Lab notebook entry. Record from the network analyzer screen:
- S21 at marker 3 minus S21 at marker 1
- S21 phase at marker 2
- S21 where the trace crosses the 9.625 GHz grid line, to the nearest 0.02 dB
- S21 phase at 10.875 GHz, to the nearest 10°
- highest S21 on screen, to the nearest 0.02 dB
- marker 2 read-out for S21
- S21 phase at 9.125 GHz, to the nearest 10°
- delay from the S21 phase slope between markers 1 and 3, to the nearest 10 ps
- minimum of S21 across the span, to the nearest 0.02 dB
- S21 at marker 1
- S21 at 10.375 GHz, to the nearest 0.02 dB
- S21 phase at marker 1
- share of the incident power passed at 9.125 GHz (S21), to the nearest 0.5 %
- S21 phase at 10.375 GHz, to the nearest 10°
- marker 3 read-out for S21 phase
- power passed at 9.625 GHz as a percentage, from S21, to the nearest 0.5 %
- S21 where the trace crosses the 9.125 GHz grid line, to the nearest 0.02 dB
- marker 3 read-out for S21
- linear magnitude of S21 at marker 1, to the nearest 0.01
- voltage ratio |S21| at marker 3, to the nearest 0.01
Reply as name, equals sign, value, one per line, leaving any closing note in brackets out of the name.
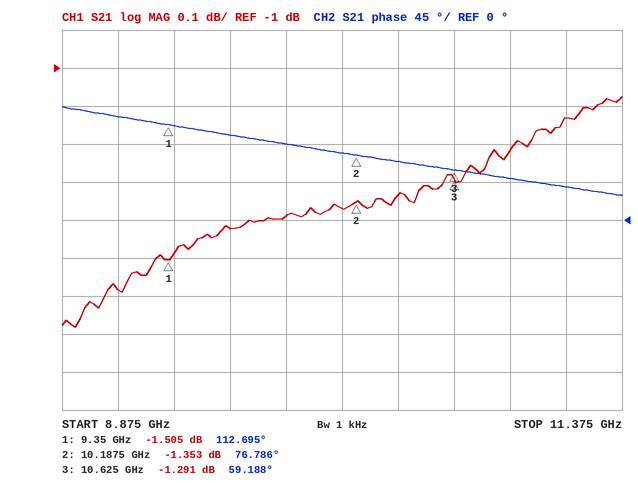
S21 at marker 3 minus S21 at marker 1 = 0.214 dB
S21 phase at marker 2 = 76.786°
S21 where the trace crosses the 9.625 GHz grid line, to the nearest 0.02 dB = -1.42 dB
S21 phase at 10.875 GHz, to the nearest 10° = 50°
highest S21 on screen, to the nearest 0.02 dB = -1.08 dB
marker 2 read-out for S21 = -1.353 dB
S21 phase at 9.125 GHz, to the nearest 10° = 120°
delay from the S21 phase slope between markers 1 and 3, to the nearest 10 ps = 120 ps
minimum of S21 across the span, to the nearest 0.02 dB = -1.68 dB
S21 at marker 1 = -1.505 dB
S21 at 10.375 GHz, to the nearest 0.02 dB = -1.34 dB
S21 phase at marker 1 = 112.695°
share of the incident power passed at 9.125 GHz (S21), to the nearest 0.5 % = 69.5 %
S21 phase at 10.375 GHz, to the nearest 10° = 70°
marker 3 read-out for S21 phase = 59.188°
power passed at 9.625 GHz as a percentage, from S21, to the nearest 0.5 % = 72.0 %
S21 where the trace crosses the 9.125 GHz grid line, to the nearest 0.02 dB = -1.58 dB
marker 3 read-out for S21 = -1.291 dB
linear magnitude of S21 at marker 1, to the nearest 0.01 = 0.84
voltage ratio |S21| at marker 3, to the nearest 0.01 = 0.86
